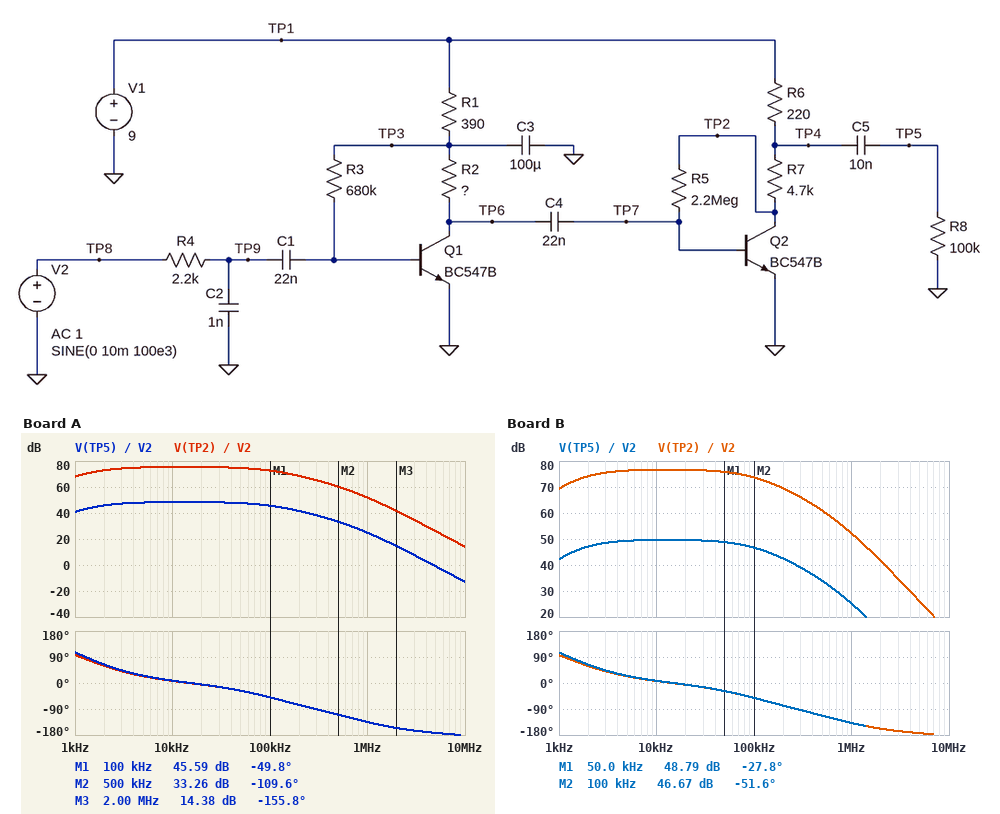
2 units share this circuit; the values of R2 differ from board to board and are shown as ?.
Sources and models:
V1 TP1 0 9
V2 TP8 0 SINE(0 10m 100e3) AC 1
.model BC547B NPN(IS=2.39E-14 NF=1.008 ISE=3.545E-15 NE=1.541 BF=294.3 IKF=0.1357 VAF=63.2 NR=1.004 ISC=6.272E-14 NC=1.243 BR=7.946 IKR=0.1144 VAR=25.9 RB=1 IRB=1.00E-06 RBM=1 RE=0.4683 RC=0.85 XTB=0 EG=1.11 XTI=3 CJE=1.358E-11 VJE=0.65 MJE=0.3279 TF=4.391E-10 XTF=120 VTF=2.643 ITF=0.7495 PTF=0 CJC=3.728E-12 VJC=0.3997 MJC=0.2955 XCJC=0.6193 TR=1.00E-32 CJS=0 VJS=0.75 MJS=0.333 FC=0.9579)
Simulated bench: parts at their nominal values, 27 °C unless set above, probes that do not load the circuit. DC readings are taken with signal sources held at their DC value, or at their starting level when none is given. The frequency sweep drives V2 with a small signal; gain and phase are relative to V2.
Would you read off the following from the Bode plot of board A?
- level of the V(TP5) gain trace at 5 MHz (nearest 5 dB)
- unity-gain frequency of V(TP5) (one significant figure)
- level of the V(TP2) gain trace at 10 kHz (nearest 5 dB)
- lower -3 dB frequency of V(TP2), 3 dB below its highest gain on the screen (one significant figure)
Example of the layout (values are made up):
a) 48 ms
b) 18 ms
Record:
a) 0 dB
b) 5 MHz
c) 75 dB
d) 2 kHz
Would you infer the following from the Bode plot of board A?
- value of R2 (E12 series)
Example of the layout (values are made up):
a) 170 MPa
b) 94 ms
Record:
a) 1 kΩ
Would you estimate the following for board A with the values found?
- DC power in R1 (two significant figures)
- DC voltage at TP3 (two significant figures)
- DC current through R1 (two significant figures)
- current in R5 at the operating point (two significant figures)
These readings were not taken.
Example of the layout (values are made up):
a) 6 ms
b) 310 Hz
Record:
a) 3.8 mW
b) 7.8 V
c) 3.1 mA
d) 2.3 µA
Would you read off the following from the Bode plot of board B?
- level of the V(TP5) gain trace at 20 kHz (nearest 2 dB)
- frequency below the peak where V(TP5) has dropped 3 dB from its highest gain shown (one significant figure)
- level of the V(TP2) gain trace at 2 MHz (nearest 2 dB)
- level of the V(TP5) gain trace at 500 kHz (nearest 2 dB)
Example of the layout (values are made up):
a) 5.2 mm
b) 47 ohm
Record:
a) 50 dB
b) 2 kHz
c) 42 dB
d) 34 dB
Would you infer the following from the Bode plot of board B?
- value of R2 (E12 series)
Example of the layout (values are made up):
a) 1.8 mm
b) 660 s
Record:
a) 1.2 kΩ
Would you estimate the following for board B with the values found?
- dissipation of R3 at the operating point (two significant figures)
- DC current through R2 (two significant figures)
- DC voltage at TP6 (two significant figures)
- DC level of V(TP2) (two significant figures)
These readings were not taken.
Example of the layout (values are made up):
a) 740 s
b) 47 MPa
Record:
a) 75 µW
b) 3.1 mA
c) 4.1 V
d) 5.6 V
